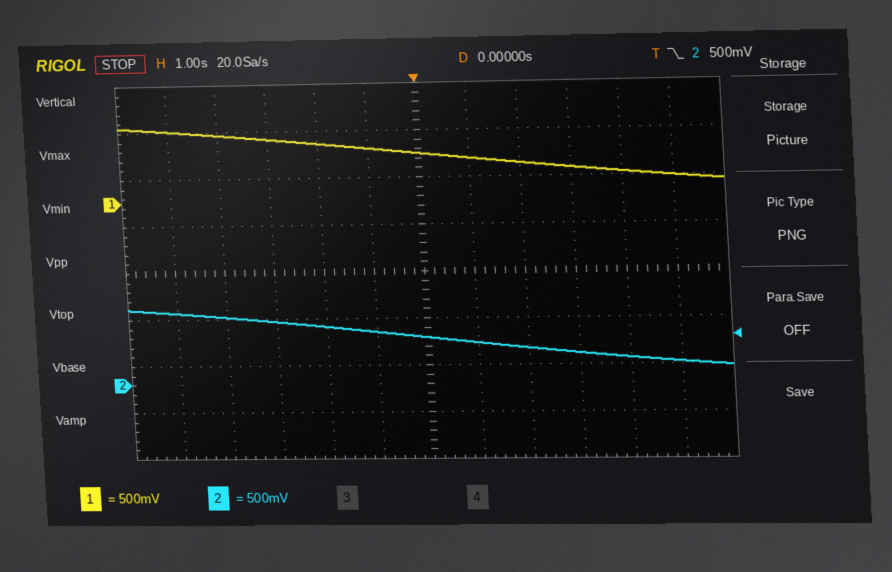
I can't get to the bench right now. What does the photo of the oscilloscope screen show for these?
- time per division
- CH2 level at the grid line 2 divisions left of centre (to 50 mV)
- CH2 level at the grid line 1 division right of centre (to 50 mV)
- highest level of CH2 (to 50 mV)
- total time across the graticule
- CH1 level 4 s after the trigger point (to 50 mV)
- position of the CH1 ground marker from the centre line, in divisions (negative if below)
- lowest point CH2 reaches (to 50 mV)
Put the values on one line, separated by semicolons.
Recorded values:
1 s; 600 mV; 450 mV; 800 mV; 12 s; 300 mV; +1.5 div; 200 mV
